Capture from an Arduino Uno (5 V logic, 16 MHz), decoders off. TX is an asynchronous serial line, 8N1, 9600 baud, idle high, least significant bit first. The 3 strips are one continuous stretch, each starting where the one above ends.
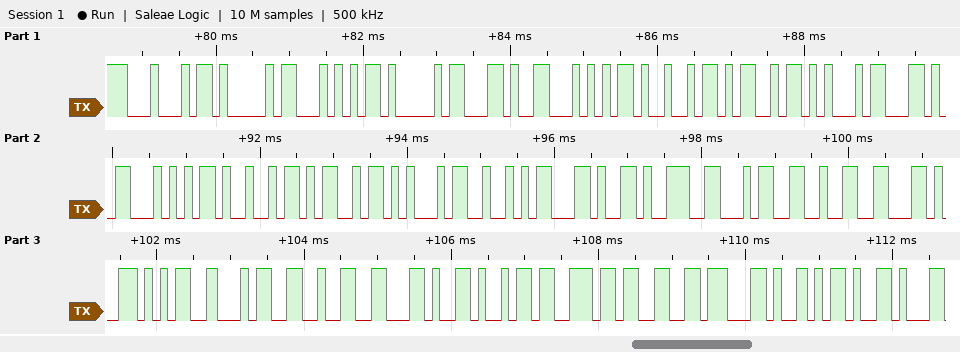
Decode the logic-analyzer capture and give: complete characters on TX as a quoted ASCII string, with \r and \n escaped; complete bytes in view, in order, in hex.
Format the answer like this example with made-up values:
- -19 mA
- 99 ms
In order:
- "DATA,TIME,TIMER,942,542,inf,-"
- 0x44 0x41 0x54 0x41 0x2C 0x54 0x49 0x4D 0x45 0x2C 0x54 0x49 0x4D 0x45 0x52 0x2C 0x39 0x34 0x32 0x2C 0x35 0x34 0x32 0x2C 0x69 0x6E 0x66 0x2C 0x2D
